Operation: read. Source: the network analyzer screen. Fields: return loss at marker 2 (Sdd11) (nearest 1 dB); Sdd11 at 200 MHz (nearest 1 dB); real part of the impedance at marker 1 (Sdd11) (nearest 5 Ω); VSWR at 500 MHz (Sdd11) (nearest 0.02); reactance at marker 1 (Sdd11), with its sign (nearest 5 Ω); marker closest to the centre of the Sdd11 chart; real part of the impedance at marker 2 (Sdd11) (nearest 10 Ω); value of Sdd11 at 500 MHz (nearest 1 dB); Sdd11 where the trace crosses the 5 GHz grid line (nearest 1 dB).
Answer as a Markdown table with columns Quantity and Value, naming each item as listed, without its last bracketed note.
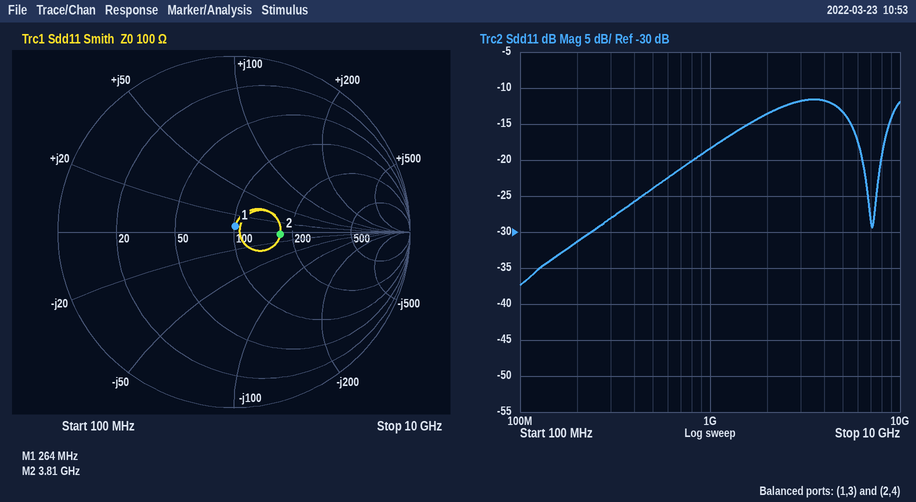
| Quantity | Value |
|---|---|
| return loss at marker 2 (Sdd11) | 12 dB |
| Sdd11 at 200 MHz | -31 dB |
| real part of the impedance at marker 1 (Sdd11) | 100 Ω |
| VSWR at 500 MHz (Sdd11) | 1.14 |
| reactance at marker 1 (Sdd11), with its sign | +5 Ω |
| marker closest to the centre of the Sdd11 chart | marker 1 |
| real part of the impedance at marker 2 (Sdd11) | 170 Ω |
| value of Sdd11 at 500 MHz | -24 dB |
| Sdd11 where the trace crosses the 5 GHz grid line | -13 dB |
